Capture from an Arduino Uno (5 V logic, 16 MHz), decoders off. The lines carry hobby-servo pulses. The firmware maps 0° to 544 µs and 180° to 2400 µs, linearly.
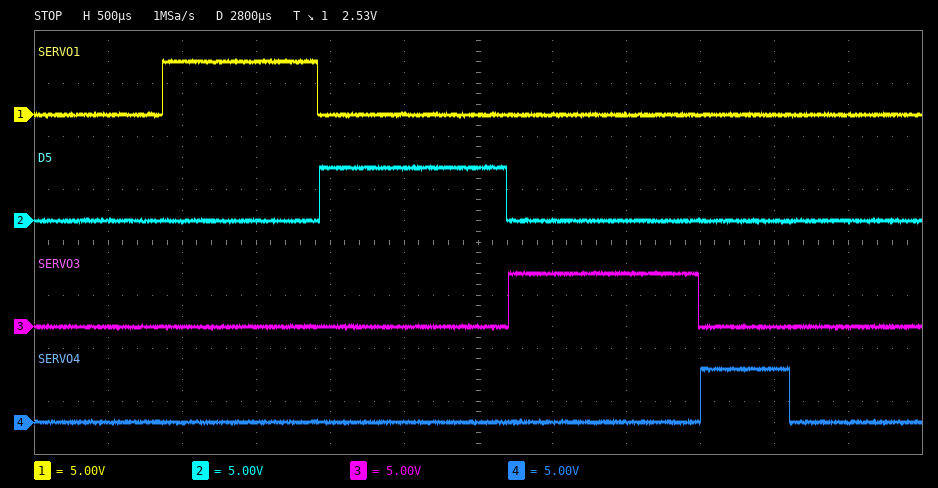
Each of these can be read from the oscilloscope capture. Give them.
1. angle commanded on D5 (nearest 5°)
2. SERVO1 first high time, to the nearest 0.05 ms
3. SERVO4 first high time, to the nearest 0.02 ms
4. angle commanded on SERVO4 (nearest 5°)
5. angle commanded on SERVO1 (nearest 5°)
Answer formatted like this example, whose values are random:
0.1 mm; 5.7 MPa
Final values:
70°; 1.05 ms; 0.60 ms; 5°; 50°
